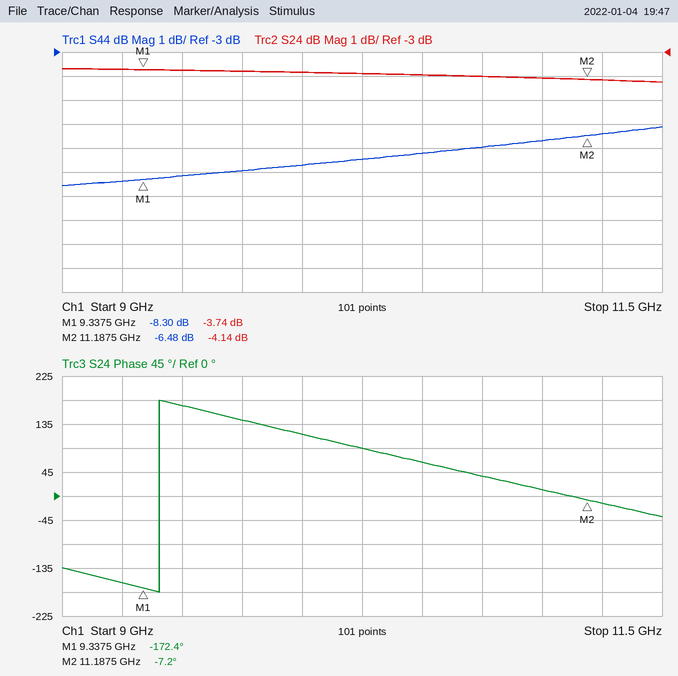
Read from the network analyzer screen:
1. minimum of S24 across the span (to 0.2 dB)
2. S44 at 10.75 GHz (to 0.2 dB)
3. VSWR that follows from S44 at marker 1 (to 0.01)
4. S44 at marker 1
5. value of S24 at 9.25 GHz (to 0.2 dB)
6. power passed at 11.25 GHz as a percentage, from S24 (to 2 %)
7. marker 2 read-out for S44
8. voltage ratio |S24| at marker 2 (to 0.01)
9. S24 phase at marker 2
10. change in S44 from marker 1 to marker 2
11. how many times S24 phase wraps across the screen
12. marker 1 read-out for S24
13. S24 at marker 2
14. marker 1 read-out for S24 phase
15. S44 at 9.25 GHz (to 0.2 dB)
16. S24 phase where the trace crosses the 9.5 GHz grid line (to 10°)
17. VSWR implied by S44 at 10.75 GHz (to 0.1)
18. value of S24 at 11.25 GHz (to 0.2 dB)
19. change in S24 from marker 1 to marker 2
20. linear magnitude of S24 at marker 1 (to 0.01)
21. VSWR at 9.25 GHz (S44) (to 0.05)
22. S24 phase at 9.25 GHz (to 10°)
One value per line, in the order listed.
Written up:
-4.2 dB
-7.0 dB
2.25
-8.30 dB
-3.8 dB
38 %
-6.48 dB
0.62
-7.2°
1.82 dB
1
-3.74 dB
-4.14 dB
-172.4°
-8.4 dB
170°
2.6
-4.2 dB
-0.40 dB
0.65
2.25
-160°
